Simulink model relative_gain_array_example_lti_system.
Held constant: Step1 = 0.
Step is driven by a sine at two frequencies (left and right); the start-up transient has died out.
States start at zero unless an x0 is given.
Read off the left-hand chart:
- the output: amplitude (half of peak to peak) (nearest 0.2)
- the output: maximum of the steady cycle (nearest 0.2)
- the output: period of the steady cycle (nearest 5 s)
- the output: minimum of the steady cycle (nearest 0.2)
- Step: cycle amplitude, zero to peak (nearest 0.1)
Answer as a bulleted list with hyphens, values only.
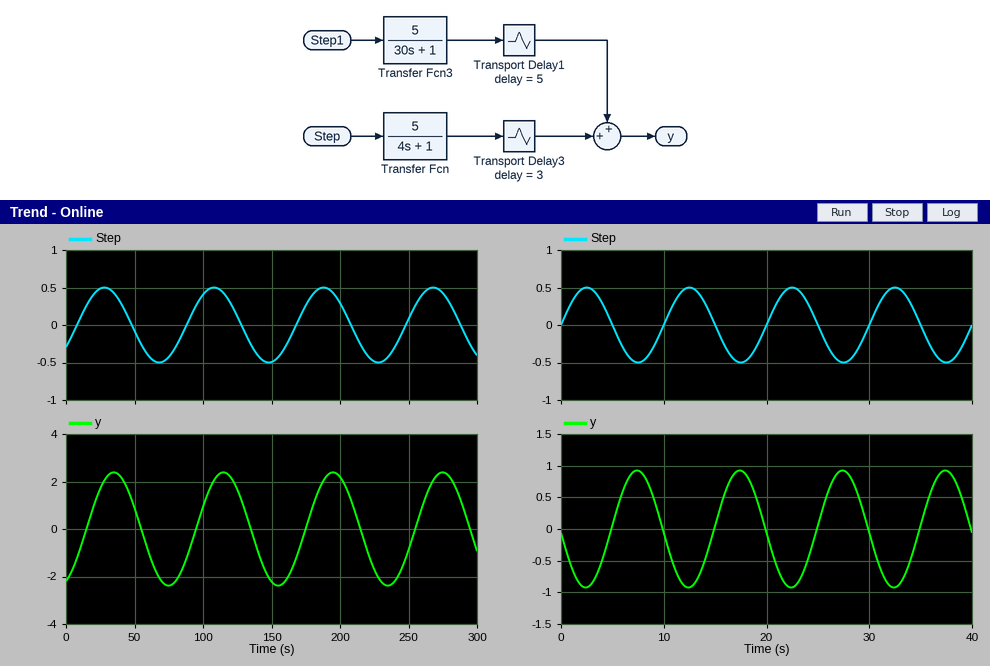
- 2.4
- 2.4
- 80 s
- -2.4
- 0.5
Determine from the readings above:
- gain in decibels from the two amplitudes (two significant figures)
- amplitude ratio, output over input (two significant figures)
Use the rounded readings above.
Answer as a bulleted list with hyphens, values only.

- 14 dB
- 4.8
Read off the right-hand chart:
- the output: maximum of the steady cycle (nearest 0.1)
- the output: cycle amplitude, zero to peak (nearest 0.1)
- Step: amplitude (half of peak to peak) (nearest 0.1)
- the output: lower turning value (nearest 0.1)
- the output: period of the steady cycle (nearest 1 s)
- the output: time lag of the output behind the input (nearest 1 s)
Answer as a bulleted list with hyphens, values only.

- 0.9
- 0.9
- 0.5
- -0.9
- 10 s
- 5 s
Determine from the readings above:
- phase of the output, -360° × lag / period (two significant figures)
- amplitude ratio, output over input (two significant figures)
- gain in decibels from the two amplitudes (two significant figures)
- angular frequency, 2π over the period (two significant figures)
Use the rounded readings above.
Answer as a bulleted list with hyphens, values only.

- -180°
- 1.8
- 5.1 dB
- 0.63 rad/s
